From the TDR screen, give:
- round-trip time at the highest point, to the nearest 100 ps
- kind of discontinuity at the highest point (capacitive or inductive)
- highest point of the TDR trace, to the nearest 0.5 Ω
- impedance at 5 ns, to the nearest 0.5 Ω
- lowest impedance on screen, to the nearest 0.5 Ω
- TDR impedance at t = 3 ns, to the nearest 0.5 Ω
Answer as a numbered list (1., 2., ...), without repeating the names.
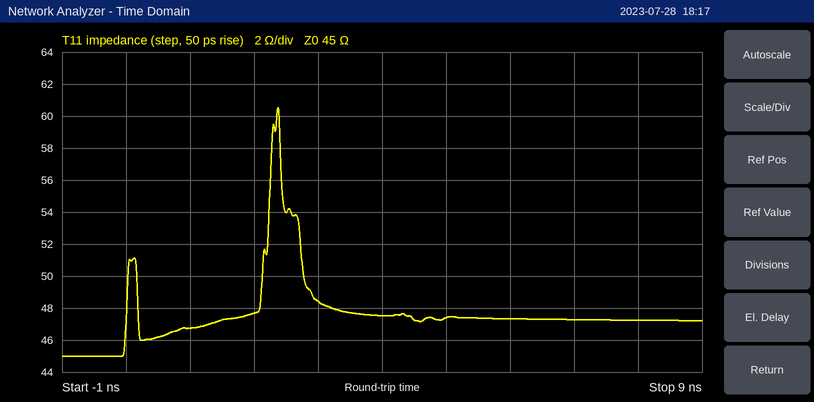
1. 2.4 ns
2. inductive
3. 60.5 Ω
4. 47.5 Ω
5. 45.0 Ω
6. 48.5 Ω
